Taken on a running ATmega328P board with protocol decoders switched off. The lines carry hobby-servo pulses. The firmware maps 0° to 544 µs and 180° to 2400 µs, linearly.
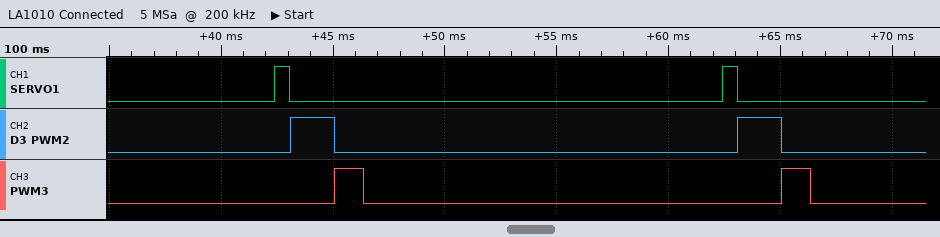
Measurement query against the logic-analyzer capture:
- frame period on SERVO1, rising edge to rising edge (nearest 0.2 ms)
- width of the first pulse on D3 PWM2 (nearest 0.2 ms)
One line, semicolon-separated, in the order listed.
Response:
20.0 ms; 2.0 ms
